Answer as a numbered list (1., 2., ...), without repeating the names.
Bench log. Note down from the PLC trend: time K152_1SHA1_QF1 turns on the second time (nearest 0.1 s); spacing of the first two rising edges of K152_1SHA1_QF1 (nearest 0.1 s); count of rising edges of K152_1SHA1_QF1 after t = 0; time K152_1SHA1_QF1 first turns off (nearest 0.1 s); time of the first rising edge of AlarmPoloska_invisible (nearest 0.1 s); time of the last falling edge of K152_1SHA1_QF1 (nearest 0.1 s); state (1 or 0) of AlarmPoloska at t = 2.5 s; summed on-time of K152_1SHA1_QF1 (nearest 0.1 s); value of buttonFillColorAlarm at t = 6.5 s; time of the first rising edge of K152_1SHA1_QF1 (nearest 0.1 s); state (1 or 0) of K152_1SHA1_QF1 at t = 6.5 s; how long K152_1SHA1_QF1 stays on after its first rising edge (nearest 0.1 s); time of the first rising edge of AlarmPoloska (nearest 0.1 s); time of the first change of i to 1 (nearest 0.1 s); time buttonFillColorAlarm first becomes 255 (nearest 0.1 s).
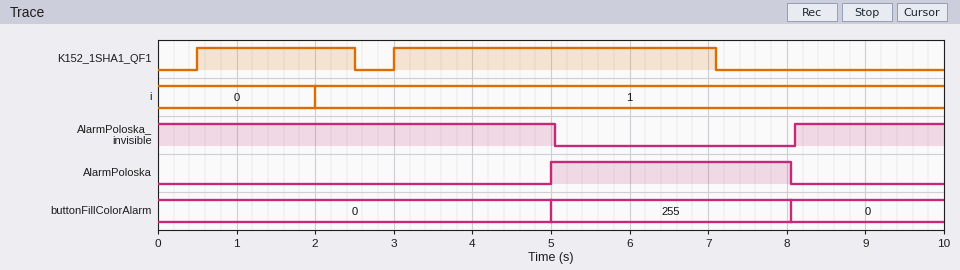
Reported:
1. 3.0 s
2. 2.5 s
3. 2
4. 2.5 s
5. 8.1 s
6. 7.1 s
7. 0
8. 6.1 s
9. 255
10. 0.5 s
11. 1
12. 2.0 s
13. 5.0 s
14. 2.0 s
15. 5.0 s
